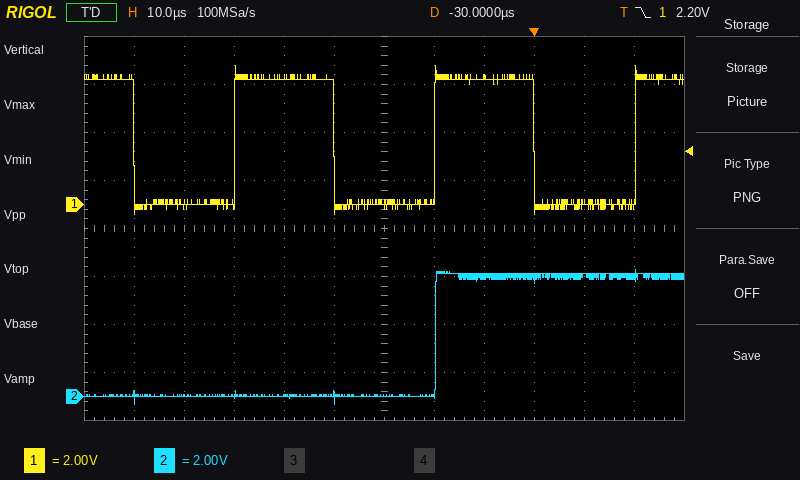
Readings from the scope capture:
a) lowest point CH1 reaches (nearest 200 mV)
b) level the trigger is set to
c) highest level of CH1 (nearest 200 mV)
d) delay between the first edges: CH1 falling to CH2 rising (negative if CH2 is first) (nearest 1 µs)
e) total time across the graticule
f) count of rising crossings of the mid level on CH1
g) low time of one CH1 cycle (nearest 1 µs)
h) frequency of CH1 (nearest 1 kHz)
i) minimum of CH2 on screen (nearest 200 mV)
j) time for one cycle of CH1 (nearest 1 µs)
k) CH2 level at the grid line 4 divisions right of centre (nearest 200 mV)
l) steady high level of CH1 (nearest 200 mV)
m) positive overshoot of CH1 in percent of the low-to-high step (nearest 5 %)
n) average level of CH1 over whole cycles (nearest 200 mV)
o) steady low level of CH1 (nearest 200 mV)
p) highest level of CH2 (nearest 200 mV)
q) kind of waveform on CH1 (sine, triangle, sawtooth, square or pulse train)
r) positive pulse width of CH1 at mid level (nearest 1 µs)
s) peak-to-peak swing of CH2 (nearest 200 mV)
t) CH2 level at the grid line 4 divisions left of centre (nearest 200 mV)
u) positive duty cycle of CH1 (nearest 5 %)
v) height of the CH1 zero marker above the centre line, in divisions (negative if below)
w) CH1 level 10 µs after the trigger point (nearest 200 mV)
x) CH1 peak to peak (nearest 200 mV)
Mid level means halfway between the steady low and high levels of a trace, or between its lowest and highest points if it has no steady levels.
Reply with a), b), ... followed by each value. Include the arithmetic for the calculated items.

a) -400 mV
b) 2.20 V
c) 5.8 V
d) +60 µs
e) 120 µs
f) 3
g) 20 µs
h) 1 / 40 µs ≈ 25 kHz
i) -400 mV
j) 40 µs
k) 5.0 V
l) 5.2 V
m) 10 %
n) 0.0 V + 0.5 × (5.2 V − (0.0 V)) ≈ 2.6 V
o) 0.0 V
p) 5.2 V
q) square
r) 20 µs
s) 5.2 V − (-400 mV) = 5.6 V
t) 0.0 V
u) 20 µs / 40 µs ≈ 50 %
v) +0.5 div
w) 0.0 V
x) 5.8 V − (-400 mV) = 6.2 V
